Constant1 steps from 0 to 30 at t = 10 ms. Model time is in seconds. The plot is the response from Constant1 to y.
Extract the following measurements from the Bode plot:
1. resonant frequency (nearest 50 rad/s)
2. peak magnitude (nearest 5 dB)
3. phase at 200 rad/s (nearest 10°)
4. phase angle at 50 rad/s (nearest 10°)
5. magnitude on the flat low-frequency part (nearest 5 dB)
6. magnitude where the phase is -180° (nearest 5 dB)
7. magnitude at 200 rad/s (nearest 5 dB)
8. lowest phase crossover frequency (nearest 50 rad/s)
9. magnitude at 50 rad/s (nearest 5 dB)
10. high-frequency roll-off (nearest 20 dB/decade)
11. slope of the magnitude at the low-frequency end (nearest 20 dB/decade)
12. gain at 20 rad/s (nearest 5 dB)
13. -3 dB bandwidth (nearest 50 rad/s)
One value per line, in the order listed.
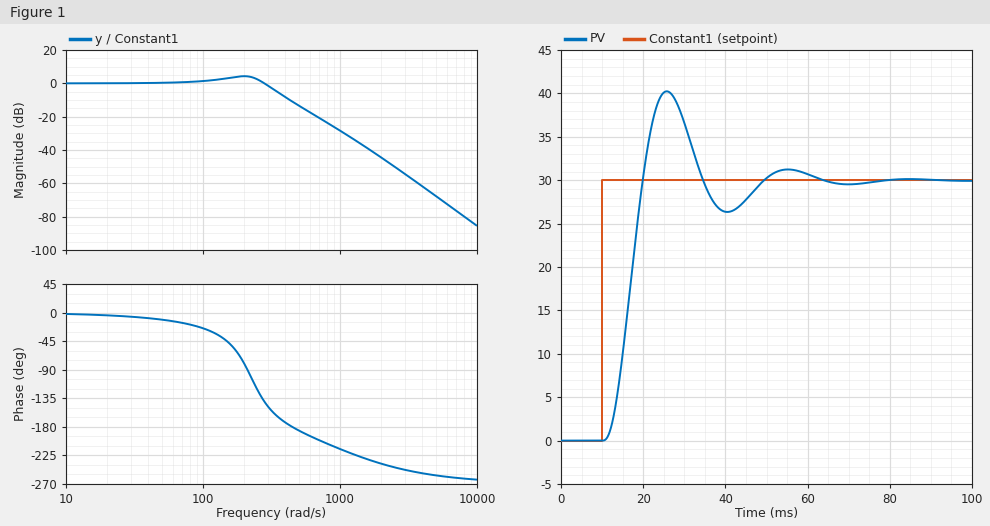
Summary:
200 rad/s
5 dB
-80°
-10°
0 dB
-10 dB
5 dB
450 rad/s
0 dB
-60 dB/decade
0 dB/decade
0 dB
300 rad/s
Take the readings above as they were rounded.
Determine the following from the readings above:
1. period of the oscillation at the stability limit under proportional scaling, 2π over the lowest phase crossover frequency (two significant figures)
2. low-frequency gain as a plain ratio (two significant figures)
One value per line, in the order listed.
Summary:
0.014 s
1.0
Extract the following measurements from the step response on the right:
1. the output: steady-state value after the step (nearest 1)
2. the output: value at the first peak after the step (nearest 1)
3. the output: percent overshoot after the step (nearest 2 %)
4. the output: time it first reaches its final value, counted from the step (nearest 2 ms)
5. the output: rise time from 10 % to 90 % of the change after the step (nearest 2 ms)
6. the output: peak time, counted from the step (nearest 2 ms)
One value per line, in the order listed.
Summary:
30
40
34 %
10 ms
6 ms
16 ms
